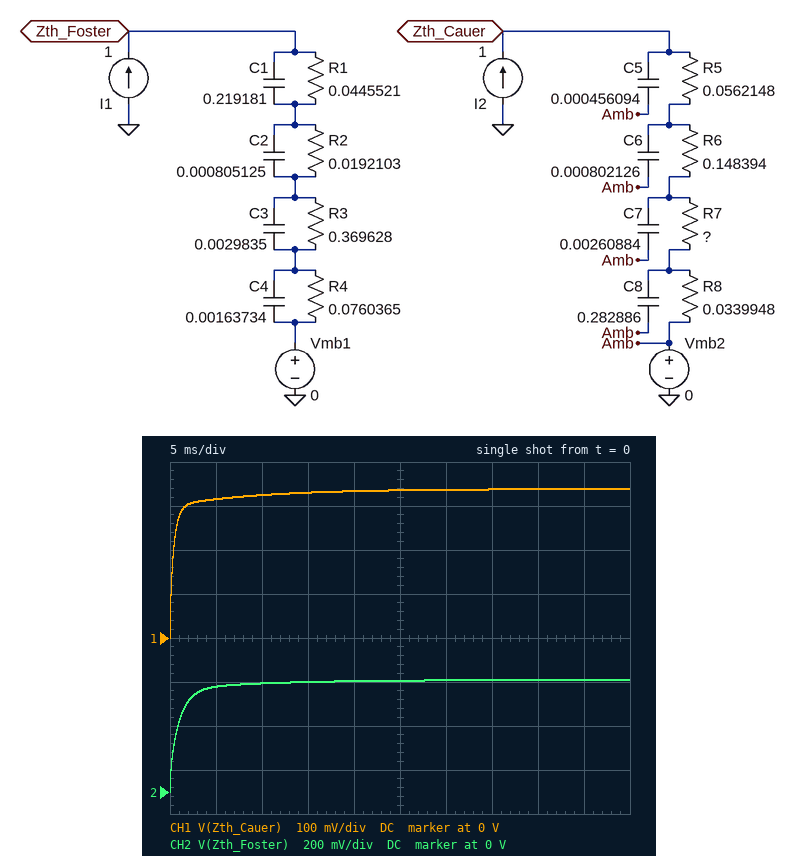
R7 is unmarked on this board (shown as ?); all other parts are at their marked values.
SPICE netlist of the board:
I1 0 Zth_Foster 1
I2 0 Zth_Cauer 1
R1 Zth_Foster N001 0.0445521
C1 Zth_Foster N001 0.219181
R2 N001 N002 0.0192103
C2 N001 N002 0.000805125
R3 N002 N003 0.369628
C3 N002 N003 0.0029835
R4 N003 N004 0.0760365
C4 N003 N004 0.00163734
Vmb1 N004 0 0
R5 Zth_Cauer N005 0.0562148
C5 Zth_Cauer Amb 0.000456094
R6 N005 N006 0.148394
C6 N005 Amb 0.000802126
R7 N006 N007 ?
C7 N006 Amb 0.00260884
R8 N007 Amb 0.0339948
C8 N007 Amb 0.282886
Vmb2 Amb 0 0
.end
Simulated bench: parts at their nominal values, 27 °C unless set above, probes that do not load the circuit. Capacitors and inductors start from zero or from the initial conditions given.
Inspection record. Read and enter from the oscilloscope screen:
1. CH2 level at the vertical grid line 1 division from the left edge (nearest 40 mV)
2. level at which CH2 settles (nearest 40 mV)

480 mV
520 mV
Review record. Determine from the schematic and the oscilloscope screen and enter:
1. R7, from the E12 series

0.1 Ω
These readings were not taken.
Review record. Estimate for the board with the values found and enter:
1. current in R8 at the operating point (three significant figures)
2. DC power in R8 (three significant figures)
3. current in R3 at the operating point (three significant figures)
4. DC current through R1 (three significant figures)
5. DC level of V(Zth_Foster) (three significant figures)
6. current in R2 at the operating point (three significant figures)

1.00 A
34.0 mW
1.00 A
1.00 A
509 mV
1.00 A
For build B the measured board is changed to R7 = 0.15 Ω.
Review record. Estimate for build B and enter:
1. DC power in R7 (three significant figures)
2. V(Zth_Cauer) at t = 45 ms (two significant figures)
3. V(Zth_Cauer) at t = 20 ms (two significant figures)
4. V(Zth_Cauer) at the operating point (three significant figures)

150 mW
390 mV
380 mV
389 mV
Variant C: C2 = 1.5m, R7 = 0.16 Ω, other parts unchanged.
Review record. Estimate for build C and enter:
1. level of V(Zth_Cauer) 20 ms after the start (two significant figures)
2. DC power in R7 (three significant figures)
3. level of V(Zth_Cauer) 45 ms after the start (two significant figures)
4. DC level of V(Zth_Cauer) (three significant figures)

390 mV
160 mW
400 mV
399 mV
